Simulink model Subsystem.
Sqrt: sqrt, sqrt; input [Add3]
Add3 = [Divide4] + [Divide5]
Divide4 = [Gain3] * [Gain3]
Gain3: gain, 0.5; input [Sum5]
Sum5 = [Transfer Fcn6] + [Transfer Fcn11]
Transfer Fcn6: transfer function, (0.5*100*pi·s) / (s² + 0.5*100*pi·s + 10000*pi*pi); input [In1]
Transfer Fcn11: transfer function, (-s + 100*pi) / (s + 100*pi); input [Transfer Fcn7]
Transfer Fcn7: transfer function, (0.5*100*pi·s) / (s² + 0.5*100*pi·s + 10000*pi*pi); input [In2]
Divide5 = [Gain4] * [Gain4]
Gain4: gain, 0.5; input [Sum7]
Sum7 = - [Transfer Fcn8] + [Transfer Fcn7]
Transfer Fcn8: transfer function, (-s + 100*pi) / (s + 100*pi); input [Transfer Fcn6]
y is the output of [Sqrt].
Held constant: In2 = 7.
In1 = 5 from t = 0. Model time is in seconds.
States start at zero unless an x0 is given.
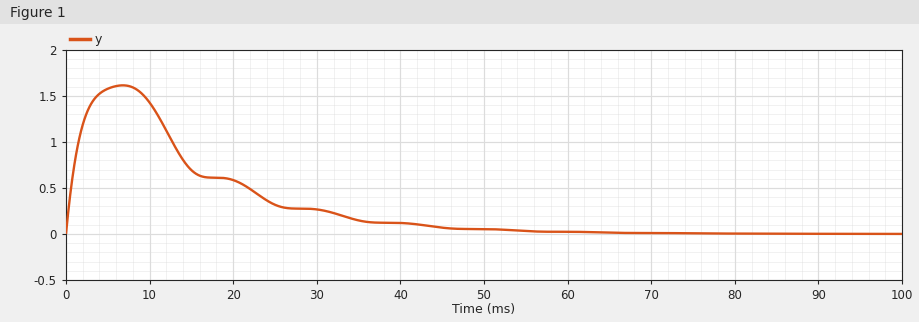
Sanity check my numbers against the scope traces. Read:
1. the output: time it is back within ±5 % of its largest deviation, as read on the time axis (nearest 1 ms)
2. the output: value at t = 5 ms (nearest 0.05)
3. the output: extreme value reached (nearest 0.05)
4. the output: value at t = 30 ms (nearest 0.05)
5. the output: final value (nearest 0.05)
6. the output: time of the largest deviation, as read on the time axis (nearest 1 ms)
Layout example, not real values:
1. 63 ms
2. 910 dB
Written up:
1. 44 ms
2. 1.60
3. 1.60
4. 0.25
5. 0.00
6. 7 ms
